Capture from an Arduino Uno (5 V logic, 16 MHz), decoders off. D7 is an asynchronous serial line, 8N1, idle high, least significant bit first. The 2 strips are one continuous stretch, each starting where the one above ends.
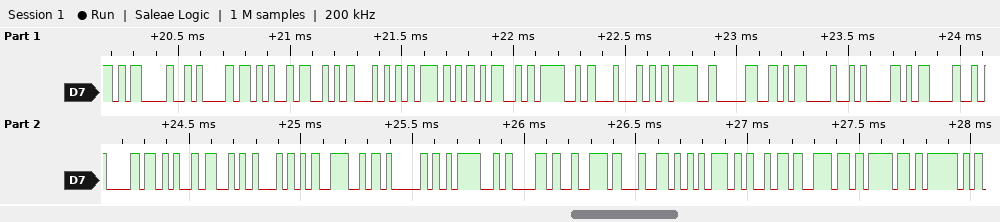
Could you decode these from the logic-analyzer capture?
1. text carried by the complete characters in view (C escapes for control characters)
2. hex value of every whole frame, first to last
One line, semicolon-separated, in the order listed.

"\r\n+STWMOD=0\r\n\r\n+STNA=arduino_"; 0x0D 0x0A 0x2B 0x53 0x54 0x57 0x4D 0x4F 0x44 0x3D 0x30 0x0D 0x0A 0x0D 0x0A 0x2B 0x53 0x54 0x4E 0x41 0x3D 0x61 0x72 0x64 0x75 0x69 0x6E 0x6F 0x5F
